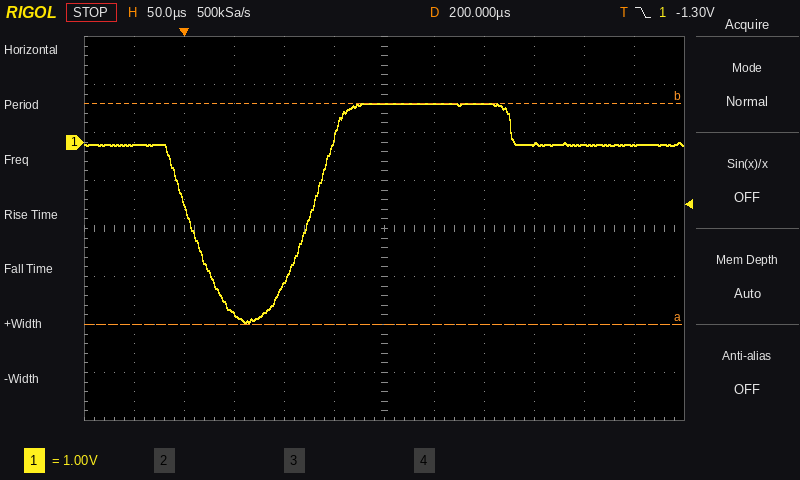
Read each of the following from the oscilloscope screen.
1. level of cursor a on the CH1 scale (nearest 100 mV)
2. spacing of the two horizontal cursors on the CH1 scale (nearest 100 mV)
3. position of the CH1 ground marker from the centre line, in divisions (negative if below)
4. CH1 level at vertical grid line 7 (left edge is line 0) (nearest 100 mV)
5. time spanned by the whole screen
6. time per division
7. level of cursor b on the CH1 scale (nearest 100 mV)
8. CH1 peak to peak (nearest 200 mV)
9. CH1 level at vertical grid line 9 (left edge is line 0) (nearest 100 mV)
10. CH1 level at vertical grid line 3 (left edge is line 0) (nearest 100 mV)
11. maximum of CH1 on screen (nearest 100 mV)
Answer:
-3.8 V
4.6 V
+1.8 div
800 mV
600 µs
50 µs
800 mV
4.6 V
0.0 V
-3.6 V
800 mV
